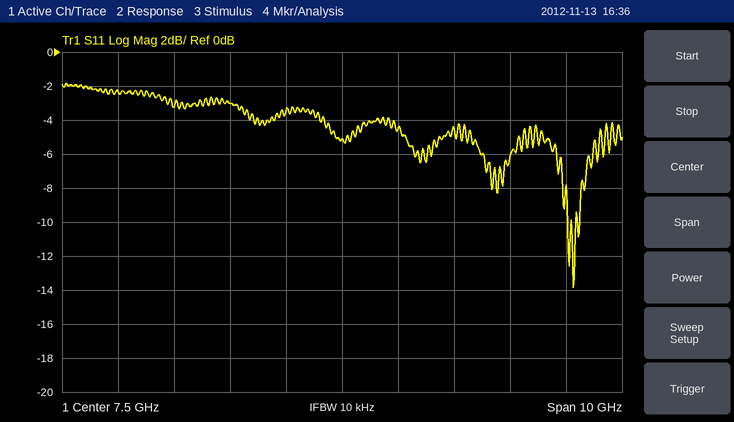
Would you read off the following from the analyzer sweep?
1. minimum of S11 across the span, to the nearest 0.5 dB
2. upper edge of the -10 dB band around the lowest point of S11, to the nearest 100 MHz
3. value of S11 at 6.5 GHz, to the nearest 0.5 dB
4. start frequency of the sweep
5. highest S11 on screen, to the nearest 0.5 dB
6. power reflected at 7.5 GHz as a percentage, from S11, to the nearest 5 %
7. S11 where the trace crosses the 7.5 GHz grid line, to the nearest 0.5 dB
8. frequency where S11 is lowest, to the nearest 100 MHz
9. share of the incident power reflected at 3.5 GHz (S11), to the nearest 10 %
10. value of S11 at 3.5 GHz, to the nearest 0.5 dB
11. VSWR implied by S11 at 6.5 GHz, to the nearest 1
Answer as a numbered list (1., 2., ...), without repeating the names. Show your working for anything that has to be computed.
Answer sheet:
1. -14.0 dB
2. 11.7 GHz
3. -3.5 dB
4. 2.5 GHz
5. -2.0 dB
6. 10^(-5/10) ≈ 31.6 %, so 30 % to the nearest 5 %
7. -5.0 dB
8. 11.6 GHz
9. 10^(-2.5/10) ≈ 56.2 %, so 60 % to the nearest 10 %
10. -2.5 dB
11. |Γ| = 10^(-3.5/20) = 0.6683; VSWR = (1 + 0.6683)/(1 − 0.6683) ≈ 5
